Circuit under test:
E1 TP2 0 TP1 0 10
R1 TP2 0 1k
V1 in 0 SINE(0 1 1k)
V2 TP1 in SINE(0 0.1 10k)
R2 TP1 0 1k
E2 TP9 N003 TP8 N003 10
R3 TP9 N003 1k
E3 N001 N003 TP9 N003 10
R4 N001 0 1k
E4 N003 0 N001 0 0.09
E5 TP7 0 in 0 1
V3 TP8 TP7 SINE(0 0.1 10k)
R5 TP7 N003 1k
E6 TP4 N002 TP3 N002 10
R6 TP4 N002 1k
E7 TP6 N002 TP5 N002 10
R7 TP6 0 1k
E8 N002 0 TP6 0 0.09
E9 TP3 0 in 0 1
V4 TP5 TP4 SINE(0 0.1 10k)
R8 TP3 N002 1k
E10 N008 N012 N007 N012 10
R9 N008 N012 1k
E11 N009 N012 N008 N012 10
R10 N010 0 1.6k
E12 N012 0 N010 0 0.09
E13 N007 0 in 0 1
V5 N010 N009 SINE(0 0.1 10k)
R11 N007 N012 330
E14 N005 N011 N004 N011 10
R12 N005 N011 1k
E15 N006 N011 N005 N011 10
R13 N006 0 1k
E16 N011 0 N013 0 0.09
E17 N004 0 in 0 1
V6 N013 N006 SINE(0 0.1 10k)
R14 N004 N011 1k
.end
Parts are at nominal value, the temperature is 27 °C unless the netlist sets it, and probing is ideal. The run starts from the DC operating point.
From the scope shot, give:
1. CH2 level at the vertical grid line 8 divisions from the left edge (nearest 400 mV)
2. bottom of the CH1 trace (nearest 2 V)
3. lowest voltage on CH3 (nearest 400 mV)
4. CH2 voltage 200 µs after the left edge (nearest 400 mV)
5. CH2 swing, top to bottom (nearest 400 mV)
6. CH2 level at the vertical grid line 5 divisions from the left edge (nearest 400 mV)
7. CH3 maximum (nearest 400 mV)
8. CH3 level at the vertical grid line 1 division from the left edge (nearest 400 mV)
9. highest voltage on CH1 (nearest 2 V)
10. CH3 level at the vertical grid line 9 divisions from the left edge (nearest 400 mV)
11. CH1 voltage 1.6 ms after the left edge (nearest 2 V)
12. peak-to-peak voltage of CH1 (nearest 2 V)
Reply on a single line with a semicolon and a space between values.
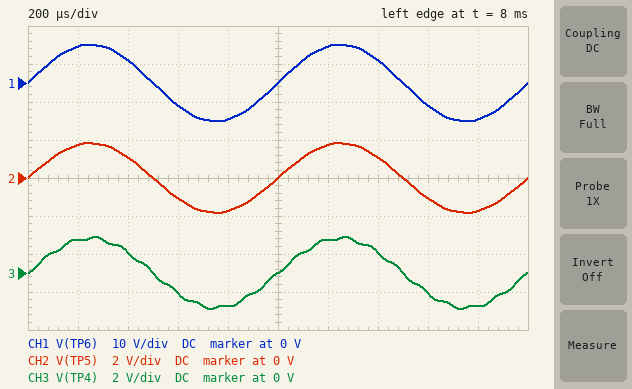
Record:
-1.2 V; -10 V; -2.0 V; 1.6 V; 3.6 V; 0 V; 2.0 V; 1.6 V; 10 V; -1.6 V; -6 V; 20 V
